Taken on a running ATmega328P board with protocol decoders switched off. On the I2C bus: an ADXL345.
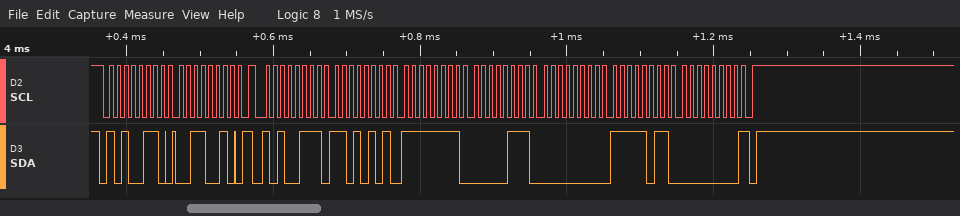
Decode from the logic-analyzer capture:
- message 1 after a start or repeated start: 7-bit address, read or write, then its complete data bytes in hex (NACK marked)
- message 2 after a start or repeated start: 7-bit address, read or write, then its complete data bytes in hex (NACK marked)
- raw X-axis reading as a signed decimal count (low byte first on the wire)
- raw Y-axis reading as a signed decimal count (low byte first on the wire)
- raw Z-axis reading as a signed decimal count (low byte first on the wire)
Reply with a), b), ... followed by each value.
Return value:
a) 0x53 write: 32
b) 0x53 read: D5 FF 07 00 FB 00 NACK
c) -43
d) 7
e) 251
